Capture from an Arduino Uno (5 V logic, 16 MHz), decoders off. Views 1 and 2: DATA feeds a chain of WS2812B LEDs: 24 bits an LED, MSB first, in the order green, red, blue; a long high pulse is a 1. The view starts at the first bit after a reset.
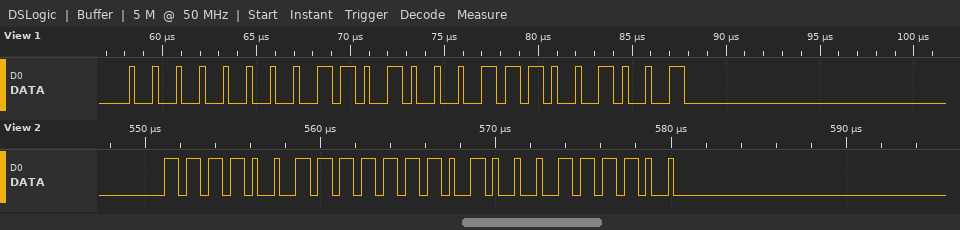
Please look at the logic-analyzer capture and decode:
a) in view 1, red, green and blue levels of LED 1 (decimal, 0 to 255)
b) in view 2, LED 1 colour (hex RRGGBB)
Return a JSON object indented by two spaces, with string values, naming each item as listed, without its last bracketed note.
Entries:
{
  "in view 1, red, green and blue levels of LED 1": "209, 0, 201",
  "in view 2, LED 1 colour": "#FAF33C"
}
